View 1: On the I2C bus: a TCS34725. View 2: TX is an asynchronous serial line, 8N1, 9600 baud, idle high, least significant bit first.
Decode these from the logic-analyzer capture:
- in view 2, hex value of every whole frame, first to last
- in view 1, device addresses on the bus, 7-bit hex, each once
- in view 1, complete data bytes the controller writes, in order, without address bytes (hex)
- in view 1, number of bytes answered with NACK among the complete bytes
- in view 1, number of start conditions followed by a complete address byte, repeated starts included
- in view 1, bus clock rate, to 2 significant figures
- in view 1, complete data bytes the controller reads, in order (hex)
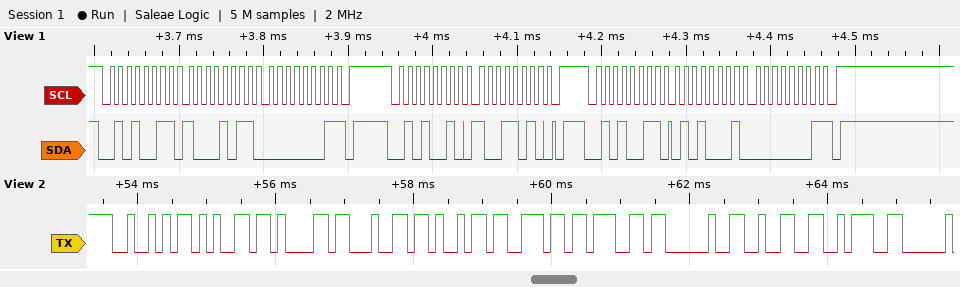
52 65 61 64 69 6E 67 20 32 3A
0x29
9A
2
3
100 kHz
8B 01 51 01
